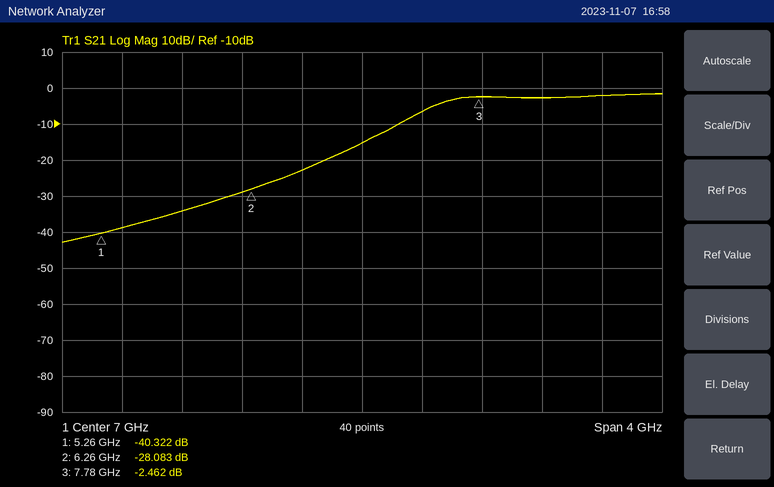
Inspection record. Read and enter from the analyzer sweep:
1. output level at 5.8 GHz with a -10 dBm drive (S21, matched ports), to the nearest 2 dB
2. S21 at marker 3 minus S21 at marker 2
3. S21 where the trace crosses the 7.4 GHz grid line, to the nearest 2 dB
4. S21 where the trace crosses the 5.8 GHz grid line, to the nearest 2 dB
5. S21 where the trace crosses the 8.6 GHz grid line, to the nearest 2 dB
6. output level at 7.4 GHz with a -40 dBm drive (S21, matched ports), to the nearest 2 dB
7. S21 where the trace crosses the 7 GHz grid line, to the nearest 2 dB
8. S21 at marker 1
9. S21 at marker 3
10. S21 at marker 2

-44 dBm
25.621 dB
-6 dB
-34 dB
-2 dB
-46 dBm
-16 dB
-40.322 dB
-2.462 dB
-28.083 dB
